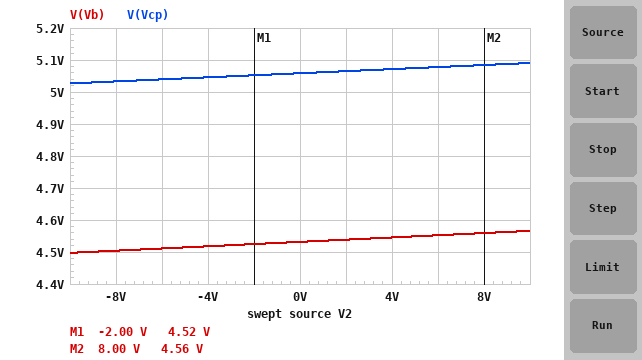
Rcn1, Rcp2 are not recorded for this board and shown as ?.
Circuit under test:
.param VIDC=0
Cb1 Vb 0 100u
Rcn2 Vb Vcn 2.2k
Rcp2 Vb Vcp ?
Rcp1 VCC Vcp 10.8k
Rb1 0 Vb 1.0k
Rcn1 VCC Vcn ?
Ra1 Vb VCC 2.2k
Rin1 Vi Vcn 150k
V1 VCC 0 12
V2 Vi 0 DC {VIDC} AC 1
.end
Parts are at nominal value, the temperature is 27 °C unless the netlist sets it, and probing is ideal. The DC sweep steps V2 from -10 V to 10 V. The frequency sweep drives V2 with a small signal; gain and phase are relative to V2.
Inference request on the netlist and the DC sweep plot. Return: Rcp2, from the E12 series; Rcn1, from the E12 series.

820 Ω
12 kΩ
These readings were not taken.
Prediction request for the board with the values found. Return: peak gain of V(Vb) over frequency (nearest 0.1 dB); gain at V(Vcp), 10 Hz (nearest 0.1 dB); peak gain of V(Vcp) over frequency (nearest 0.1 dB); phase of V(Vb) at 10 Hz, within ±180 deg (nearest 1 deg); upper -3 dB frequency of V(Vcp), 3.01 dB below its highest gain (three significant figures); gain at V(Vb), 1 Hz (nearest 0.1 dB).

-49.3 dB
-62.0 dB
-49.9 dB
-76 deg
2.57 Hz
-49.9 dB
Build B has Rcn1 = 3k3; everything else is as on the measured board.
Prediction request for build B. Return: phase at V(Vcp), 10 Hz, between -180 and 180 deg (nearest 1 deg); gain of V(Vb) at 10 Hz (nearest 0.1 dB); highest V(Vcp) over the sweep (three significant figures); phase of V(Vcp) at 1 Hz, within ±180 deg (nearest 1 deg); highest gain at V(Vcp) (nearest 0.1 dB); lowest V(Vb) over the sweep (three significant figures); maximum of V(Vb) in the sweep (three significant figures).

-75 deg
-64.3 dB
5.53 V
-20 deg
-53.4 dB
4.99 V
5.04 V
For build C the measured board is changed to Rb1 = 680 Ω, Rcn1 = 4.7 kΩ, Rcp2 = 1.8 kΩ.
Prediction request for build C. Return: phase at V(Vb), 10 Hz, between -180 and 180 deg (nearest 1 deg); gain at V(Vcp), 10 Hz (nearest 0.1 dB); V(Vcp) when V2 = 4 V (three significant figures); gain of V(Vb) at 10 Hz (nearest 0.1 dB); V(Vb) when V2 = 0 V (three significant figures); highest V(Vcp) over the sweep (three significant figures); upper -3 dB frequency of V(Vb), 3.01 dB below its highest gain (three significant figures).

-71 deg
-64.7 dB
4.96 V
-63.4 dB
3.78 V
4.97 V
3.43 Hz
